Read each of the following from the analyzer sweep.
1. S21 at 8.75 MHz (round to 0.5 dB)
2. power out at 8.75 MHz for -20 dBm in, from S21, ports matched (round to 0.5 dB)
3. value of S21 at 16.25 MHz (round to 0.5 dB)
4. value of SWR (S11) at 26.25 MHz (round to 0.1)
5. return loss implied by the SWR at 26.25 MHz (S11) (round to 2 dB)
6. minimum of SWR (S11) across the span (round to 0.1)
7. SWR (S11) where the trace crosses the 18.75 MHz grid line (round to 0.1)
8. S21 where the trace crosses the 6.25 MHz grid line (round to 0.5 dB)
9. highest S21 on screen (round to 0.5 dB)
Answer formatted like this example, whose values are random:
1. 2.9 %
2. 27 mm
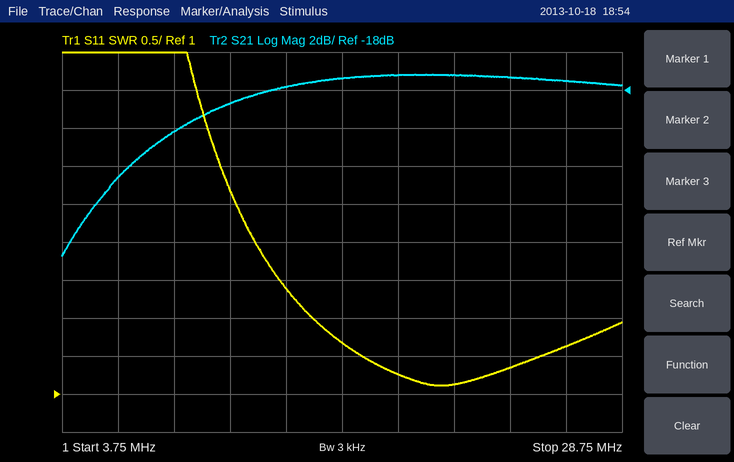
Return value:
1. -20.0 dB
2. -40.0 dBm
3. -17.5 dB
4. 1.6
5. 12 dB
6. 1.1
7. 1.3
8. -22.5 dB
9. -17.0 dB
